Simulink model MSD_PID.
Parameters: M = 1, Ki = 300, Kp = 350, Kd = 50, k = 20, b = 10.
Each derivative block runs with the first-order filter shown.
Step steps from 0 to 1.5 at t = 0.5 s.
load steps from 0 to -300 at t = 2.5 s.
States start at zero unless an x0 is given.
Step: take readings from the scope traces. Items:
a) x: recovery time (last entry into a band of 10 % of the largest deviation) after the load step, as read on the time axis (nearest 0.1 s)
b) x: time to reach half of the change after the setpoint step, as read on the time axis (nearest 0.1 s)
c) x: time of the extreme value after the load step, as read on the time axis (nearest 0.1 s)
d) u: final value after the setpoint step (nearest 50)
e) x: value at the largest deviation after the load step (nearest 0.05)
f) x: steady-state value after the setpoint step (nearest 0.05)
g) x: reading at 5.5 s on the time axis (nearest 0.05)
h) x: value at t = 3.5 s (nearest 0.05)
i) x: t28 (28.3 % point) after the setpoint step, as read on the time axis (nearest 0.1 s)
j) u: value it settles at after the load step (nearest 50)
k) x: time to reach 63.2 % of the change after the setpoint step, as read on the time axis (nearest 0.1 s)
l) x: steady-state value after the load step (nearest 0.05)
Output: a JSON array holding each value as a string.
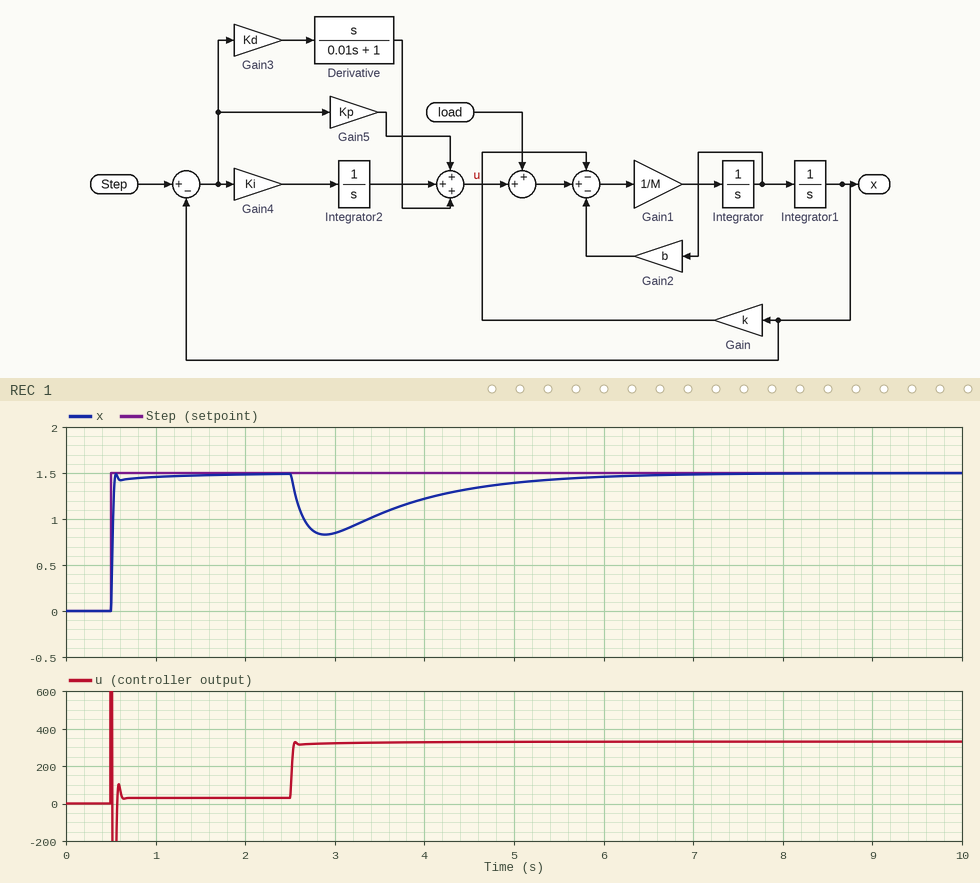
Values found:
["5.5 s", "0.5 s", "2.9 s", "50", "0.85", "1.50", "1.45", "1.05", "0.5 s", "350", "0.5 s", "1.50"]
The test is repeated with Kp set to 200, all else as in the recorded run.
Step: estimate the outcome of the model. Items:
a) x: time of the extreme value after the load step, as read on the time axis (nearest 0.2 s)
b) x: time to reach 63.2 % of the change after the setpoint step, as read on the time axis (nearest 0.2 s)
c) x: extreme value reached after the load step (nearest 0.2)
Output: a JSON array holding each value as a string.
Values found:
["3.0 s", "0.6 s", "0.6"]
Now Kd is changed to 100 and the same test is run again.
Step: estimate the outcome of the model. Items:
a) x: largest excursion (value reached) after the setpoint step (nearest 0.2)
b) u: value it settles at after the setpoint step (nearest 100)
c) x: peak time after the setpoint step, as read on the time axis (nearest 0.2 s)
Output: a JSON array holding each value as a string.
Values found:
["1.6", "0", "0.6 s"]
